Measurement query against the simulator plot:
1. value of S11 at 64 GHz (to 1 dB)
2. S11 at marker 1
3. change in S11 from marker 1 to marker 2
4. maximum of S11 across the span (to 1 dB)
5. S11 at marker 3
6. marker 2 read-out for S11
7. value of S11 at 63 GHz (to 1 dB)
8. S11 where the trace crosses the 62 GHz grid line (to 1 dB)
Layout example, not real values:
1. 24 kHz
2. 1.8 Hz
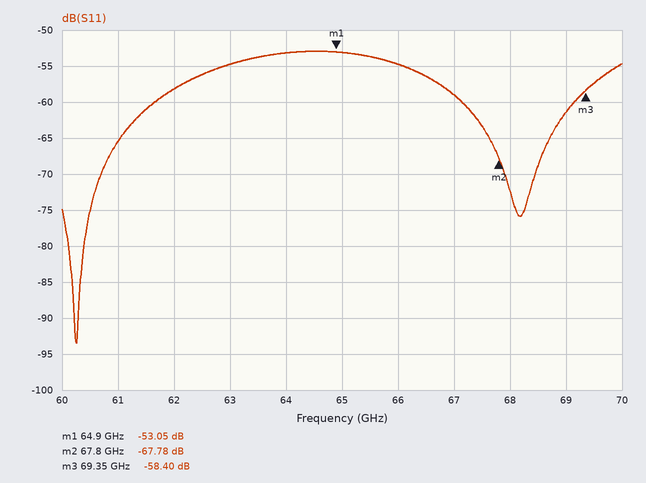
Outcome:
1. -53 dB
2. -53.05 dB
3. -14.73 dB
4. -53 dB
5. -58.40 dB
6. -67.78 dB
7. -55 dB
8. -58 dB
